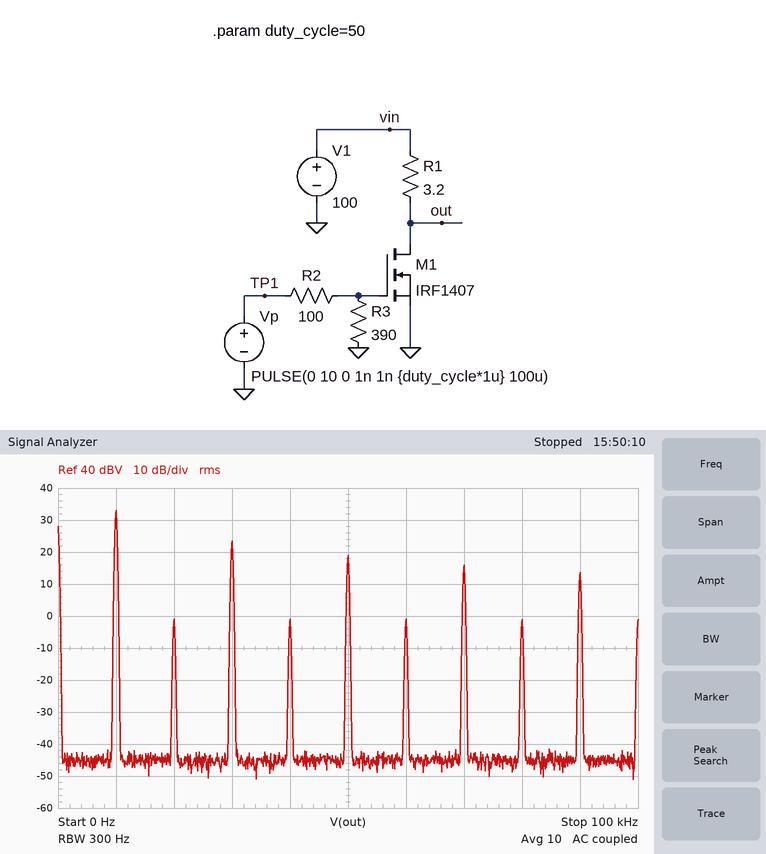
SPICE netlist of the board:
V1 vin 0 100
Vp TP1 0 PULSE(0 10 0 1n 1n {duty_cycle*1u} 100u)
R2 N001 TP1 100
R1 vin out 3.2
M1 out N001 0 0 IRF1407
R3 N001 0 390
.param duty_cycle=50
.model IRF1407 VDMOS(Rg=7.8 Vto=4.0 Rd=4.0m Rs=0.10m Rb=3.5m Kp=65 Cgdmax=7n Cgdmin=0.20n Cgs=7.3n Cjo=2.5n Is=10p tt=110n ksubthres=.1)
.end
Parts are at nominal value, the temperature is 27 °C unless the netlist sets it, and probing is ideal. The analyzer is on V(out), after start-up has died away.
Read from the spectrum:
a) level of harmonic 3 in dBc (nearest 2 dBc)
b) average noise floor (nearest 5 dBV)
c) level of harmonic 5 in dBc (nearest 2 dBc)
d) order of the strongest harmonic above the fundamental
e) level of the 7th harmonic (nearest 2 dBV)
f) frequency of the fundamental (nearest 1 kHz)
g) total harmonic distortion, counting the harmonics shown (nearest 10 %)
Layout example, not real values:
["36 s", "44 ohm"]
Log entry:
["-10 dBc", "-45 dBV", "-14 dBc", "3", "16 dBV", "10 kHz", "40 %"]
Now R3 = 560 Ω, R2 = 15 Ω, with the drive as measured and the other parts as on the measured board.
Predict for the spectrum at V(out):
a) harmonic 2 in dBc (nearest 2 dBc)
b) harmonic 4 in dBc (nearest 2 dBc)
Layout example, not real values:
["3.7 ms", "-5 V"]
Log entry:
["-40 dBc", "-40 dBc"]
